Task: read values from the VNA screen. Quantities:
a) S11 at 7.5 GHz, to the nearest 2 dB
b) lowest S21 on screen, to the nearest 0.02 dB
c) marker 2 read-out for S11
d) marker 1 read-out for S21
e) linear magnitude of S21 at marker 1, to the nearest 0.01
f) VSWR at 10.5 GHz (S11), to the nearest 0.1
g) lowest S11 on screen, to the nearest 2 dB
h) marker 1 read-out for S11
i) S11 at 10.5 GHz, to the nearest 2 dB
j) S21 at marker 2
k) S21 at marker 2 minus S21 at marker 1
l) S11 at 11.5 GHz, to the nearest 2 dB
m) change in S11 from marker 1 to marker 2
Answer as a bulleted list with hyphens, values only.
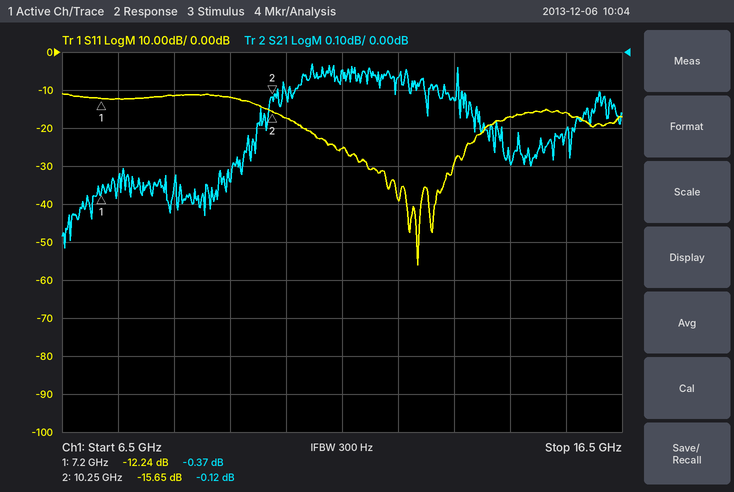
- -12 dB
- -0.52 dB
- -15.65 dB
- -0.37 dB
- 0.96
- 1.3
- -56 dB
- -12.24 dB
- -18 dB
- -0.12 dB
- 0.25 dB
- -26 dB
- -3.41 dB
